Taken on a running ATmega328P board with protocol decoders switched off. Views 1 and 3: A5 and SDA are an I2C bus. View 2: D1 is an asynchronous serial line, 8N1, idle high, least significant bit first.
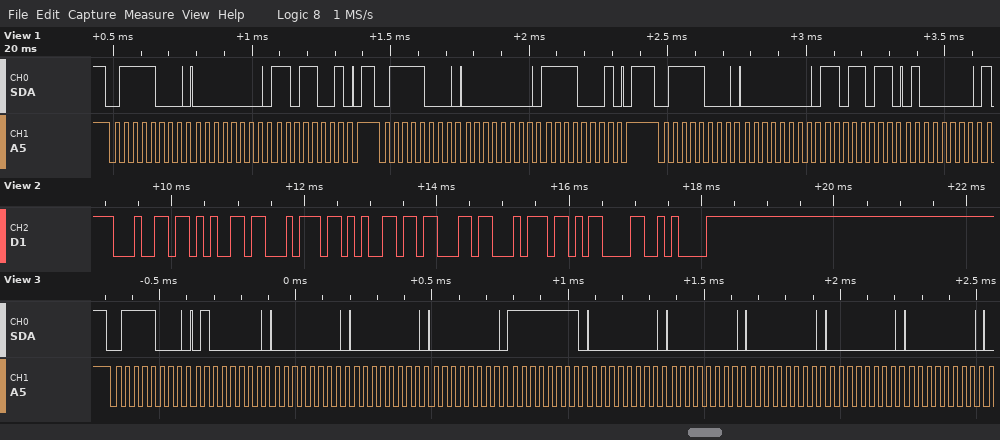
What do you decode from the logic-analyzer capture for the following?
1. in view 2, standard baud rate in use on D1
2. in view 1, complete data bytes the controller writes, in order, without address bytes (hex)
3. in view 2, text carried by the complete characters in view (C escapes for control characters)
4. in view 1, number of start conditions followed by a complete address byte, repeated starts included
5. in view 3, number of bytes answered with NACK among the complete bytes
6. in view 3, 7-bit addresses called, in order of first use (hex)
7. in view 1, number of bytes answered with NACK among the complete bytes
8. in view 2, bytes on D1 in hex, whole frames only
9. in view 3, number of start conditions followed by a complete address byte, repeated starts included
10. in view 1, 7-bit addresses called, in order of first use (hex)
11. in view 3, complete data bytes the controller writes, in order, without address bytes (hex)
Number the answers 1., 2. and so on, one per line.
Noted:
1. 9600 baud
2. 00 D9 00 F1 00 DB 40
3. "detect\r\n"
4. 3
5. 0
6. 0x3C
7. 0
8. 64 65 74 65 63 74 0D 0A
9. 1
10. 0x3C
11. 40 00 00 00 FF 00 00 00 00 00
